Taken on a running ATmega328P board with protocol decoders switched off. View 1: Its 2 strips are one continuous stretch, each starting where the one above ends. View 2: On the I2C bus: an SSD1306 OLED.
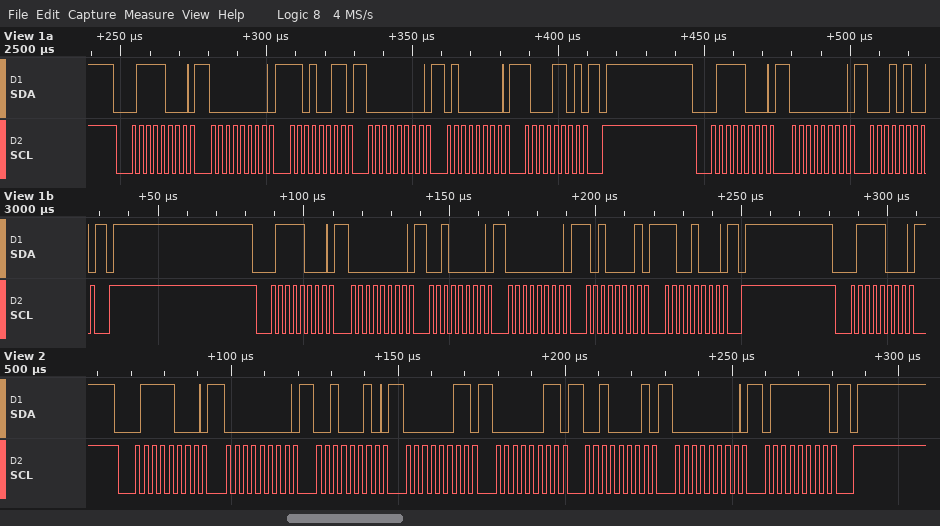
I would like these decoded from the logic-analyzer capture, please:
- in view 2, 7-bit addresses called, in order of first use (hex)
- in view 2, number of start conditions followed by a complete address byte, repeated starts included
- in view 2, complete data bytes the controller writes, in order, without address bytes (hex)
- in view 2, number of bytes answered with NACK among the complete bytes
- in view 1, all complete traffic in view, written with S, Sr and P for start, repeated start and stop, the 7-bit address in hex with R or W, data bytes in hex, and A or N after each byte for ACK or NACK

0x3C
1
00 22 03 03 21 00 7F
0
S 3CW A 00 A D3 A 00 A 40 A 8D A P S 3CW A 00 A 14 A P S 3CW A 00 A 20 A 00 A A1 A C8 A P S 3CW A
